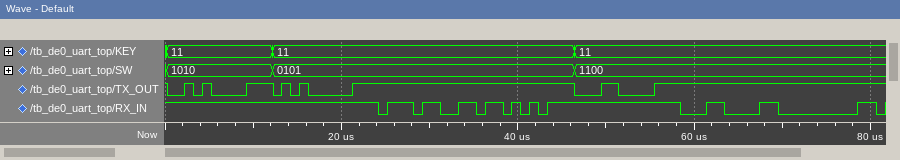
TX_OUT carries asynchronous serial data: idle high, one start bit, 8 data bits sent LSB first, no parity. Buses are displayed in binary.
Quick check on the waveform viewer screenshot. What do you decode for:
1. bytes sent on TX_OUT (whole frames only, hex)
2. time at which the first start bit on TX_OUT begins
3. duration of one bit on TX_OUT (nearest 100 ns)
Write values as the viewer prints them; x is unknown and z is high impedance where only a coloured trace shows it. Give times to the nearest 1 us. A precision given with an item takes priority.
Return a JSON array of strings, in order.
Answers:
["0A, 05, 0C", "0 us", "1000 ns"]
